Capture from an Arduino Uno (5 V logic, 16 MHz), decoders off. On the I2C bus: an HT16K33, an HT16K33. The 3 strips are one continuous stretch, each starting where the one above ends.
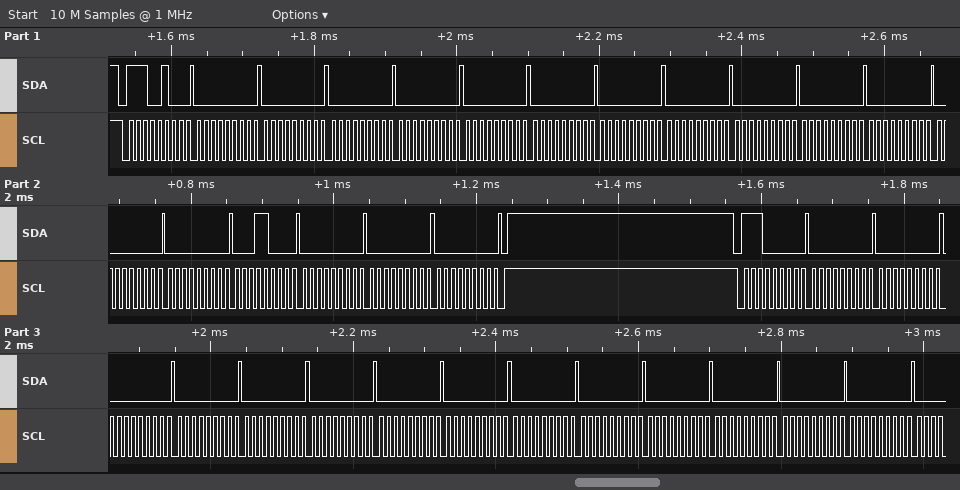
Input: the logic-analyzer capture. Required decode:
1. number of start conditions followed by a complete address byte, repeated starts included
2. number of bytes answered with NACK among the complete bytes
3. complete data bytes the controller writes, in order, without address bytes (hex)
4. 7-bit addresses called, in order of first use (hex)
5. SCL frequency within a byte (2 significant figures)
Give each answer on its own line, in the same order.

2
0
00 00 00 00 00 00 00 00 00 00 00 00 00 18 00 00 00 00 00 00 00 00 00 00 00 00 00 00 00 00 00
0x72 0x70
100 kHz
